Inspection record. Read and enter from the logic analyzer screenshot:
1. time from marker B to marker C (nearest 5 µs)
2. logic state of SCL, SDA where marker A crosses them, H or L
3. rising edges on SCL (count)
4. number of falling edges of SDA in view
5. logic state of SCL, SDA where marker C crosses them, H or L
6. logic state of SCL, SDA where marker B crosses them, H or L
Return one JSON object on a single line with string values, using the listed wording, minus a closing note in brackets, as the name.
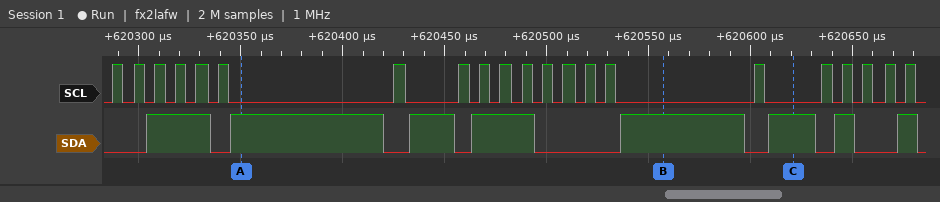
{"time from marker B to marker C": "65 µs", "logic state of SCL, SDA where marker A crosses them, H or L": "SCL=L, SDA=H", "rising edges on SCL": "21", "number of falling edges of SDA in view": "8", "logic state of SCL, SDA where marker C crosses them, H or L": "SCL=L, SDA=H", "logic state of SCL, SDA where marker B crosses them, H or L": "SCL=L, SDA=H"}
